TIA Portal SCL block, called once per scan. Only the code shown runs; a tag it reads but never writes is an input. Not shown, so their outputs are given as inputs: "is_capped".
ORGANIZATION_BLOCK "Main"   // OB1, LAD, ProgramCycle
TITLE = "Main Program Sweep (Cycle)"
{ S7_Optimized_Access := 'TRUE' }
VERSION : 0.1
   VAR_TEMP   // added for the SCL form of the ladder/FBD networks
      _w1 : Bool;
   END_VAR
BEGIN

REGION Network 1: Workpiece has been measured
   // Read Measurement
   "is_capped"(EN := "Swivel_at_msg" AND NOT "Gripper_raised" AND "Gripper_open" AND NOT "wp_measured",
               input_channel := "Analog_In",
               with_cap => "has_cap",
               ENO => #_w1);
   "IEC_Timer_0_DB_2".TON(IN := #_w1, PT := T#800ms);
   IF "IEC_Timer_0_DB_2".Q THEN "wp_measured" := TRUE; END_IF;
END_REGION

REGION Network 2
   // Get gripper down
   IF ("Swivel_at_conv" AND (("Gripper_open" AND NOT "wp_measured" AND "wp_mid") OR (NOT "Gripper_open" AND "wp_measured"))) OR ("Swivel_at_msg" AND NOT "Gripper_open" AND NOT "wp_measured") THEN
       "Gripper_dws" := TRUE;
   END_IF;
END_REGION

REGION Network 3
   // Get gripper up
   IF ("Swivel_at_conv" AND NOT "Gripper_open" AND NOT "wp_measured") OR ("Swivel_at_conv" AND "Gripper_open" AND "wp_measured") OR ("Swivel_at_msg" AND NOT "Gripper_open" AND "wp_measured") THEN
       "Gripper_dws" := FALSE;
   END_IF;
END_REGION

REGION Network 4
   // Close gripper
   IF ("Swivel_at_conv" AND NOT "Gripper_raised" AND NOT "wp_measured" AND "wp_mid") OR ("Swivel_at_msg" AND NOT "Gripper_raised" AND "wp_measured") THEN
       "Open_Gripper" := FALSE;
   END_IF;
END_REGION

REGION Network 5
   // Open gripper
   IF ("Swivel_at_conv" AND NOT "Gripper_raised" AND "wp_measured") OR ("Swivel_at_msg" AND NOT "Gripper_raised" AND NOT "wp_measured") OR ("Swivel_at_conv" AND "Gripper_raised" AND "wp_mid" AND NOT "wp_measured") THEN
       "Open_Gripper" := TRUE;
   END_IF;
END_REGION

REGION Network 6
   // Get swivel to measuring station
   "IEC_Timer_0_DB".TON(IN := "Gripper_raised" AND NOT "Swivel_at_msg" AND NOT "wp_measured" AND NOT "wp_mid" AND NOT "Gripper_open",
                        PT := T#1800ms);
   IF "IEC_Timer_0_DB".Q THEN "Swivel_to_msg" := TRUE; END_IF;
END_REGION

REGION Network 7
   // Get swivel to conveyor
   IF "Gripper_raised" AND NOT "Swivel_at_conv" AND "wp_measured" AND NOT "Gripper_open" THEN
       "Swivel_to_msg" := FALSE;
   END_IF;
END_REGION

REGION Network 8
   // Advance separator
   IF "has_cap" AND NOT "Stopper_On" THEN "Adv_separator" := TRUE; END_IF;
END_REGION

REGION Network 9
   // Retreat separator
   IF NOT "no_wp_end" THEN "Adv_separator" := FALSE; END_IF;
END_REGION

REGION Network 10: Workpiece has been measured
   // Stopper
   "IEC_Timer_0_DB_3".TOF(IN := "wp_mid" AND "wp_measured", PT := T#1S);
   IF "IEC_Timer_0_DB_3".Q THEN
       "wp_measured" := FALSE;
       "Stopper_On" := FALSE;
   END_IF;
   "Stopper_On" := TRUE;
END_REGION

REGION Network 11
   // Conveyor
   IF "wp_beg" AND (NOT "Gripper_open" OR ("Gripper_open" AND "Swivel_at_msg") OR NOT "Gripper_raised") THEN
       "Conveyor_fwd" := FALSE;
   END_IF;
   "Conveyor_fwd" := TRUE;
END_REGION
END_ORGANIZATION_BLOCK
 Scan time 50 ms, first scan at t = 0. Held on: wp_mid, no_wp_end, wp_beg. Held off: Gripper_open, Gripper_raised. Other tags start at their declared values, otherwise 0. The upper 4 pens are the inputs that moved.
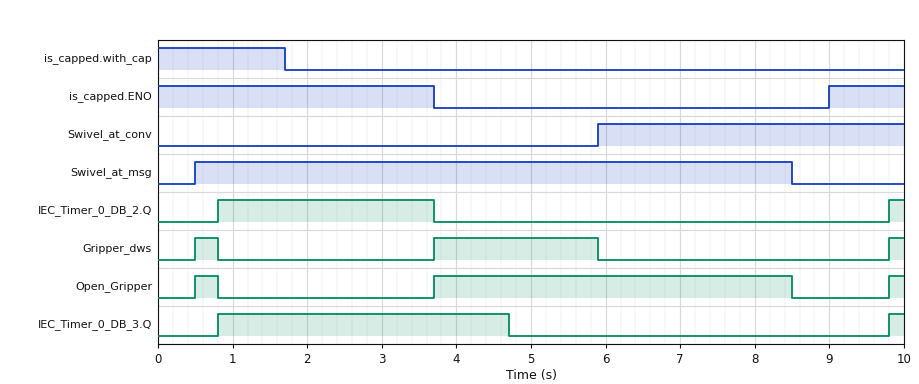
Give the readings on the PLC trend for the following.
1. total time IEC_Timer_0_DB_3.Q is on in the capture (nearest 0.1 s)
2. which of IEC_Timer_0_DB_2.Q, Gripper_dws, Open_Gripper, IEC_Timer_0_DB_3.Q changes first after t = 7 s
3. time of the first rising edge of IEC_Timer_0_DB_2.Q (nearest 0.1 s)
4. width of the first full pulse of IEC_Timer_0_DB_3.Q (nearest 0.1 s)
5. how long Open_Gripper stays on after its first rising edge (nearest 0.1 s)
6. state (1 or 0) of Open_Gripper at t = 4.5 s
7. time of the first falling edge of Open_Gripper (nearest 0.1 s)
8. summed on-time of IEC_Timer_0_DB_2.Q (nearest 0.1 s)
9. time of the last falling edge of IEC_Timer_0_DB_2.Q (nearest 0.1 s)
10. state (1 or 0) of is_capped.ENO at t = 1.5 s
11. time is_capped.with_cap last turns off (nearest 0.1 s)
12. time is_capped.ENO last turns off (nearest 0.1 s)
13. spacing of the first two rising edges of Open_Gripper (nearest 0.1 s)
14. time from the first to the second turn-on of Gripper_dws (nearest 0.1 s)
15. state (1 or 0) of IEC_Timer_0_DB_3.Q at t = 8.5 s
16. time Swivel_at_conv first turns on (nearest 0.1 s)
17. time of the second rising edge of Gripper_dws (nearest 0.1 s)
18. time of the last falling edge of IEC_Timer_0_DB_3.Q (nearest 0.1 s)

4.1 s
Open_Gripper
0.8 s
3.9 s
0.3 s
1
0.8 s
3.1 s
3.7 s
1
1.7 s
3.7 s
3.2 s
3.2 s
0
5.9 s
3.7 s
4.7 s
